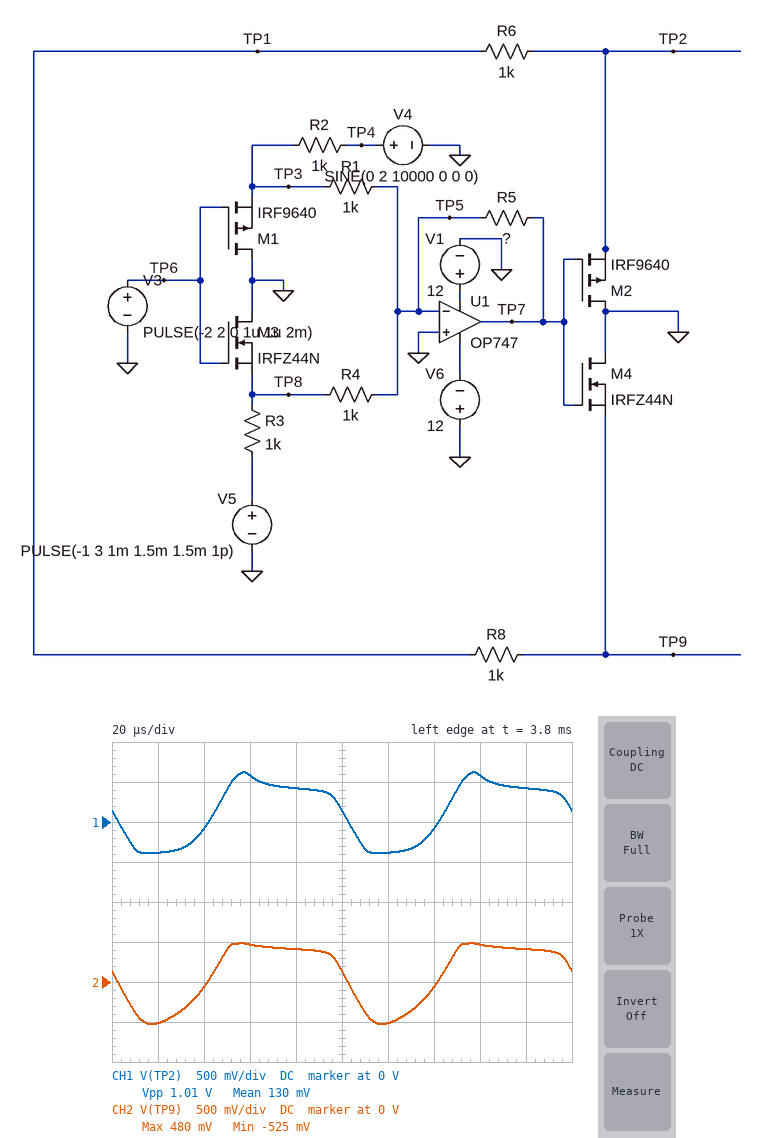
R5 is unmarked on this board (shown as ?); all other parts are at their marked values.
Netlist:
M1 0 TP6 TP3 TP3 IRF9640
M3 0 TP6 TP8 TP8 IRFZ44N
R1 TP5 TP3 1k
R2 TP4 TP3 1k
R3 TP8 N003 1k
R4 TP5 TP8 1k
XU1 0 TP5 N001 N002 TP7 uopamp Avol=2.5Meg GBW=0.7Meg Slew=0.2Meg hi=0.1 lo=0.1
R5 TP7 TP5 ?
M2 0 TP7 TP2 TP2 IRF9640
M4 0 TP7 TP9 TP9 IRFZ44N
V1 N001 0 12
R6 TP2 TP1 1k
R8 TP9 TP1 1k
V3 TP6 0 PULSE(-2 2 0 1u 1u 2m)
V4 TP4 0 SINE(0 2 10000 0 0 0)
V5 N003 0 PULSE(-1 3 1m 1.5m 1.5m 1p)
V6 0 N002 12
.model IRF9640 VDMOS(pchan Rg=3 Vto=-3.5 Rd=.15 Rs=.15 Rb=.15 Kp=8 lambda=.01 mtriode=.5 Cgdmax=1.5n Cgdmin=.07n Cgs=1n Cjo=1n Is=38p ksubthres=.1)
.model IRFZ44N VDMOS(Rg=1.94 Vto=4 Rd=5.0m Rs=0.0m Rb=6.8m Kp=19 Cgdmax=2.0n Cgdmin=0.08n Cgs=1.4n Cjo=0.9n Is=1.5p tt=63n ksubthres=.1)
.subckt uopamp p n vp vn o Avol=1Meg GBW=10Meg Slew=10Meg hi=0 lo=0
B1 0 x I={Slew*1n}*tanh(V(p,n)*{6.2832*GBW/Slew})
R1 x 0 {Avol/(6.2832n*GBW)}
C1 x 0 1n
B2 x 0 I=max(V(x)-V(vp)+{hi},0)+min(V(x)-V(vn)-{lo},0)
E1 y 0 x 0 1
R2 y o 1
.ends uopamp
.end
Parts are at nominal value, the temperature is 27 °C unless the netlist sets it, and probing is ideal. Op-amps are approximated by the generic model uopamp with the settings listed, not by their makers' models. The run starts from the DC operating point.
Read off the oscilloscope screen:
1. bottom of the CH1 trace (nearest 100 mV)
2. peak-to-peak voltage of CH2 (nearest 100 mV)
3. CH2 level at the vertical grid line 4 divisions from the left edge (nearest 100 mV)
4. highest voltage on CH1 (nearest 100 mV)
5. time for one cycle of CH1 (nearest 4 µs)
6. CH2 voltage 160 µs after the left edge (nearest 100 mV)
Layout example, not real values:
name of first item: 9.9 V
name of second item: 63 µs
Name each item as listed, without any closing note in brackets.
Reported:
bottom of the CH1 trace: -400 mV
peak-to-peak voltage of CH2: 1.0 V
CH2 level at the vertical grid line 4 divisions from the left edge: 400 mV
highest voltage on CH1: 600 mV
time for one cycle of CH1: 100 µs
CH2 voltage 160 µs after the left edge: 500 mV
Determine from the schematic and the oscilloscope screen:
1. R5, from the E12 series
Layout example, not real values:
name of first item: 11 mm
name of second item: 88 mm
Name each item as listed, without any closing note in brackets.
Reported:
R5, from the E12 series: 1.5 kΩ
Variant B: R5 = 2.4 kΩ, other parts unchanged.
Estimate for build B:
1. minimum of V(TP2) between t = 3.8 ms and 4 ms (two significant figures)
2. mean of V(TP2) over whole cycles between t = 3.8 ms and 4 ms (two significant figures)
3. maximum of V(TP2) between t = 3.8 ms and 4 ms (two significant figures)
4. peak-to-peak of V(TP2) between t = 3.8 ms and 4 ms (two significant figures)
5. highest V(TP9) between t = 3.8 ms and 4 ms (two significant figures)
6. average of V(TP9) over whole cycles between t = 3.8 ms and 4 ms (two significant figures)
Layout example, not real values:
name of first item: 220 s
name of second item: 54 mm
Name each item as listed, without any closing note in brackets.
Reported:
minimum of V(TP2) between t = 3.8 ms and 4 ms: -410 mV
mean of V(TP2) over whole cycles between t = 3.8 ms and 4 ms: 160 mV
maximum of V(TP2) between t = 3.8 ms and 4 ms: 780 mV
peak-to-peak of V(TP2) between t = 3.8 ms and 4 ms: 1.2 V
highest V(TP9) between t = 3.8 ms and 4 ms: 500 mV
average of V(TP9) over whole cycles between t = 3.8 ms and 4 ms: 64 mV
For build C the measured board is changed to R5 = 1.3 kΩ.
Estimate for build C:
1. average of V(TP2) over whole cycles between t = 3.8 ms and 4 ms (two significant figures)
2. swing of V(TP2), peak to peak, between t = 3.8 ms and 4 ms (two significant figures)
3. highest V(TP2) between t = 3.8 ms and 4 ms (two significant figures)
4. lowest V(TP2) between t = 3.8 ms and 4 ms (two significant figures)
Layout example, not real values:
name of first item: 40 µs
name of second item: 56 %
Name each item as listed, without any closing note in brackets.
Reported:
average of V(TP2) over whole cycles between t = 3.8 ms and 4 ms: 120 mV
swing of V(TP2), peak to peak, between t = 3.8 ms and 4 ms: 950 mV
highest V(TP2) between t = 3.8 ms and 4 ms: 570 mV
lowest V(TP2) between t = 3.8 ms and 4 ms: -380 mV
